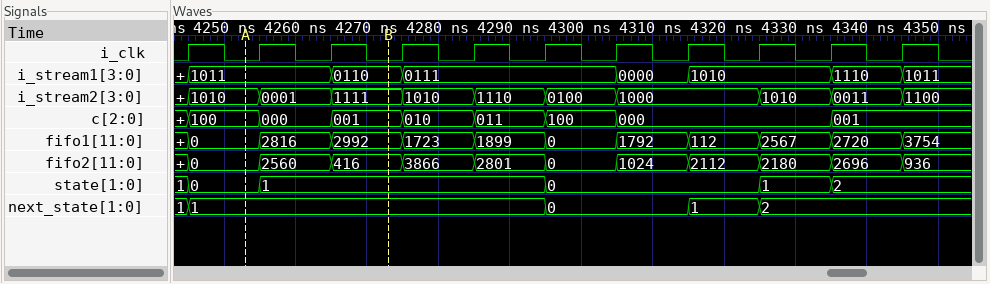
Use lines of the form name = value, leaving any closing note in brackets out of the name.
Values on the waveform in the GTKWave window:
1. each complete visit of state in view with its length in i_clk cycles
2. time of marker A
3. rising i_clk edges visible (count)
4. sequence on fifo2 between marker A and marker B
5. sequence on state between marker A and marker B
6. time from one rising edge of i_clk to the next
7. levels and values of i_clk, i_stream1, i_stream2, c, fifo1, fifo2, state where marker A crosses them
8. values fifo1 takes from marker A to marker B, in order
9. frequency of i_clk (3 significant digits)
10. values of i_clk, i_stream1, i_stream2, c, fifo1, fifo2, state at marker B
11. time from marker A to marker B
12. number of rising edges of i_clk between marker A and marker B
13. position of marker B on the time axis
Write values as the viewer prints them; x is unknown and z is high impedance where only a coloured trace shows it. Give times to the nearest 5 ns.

each complete visit of state in view with its length in i_clk cycles = 0: 1, 1: 4, 0: 3, 1: 1
time of marker A = 4255 ns
rising i_clk edges visible = 11
sequence on fifo2 between marker A and marker B = 0, 2560, 416
sequence on state between marker A and marker B = 0, 1
time from one rising edge of i_clk to the next = 10 ns
levels and values of i_clk, i_stream1, i_stream2, c, fifo1, fifo2, state where marker A crosses them = i_clk=0, i_stream1=1011, i_stream2=1010, c=100, fifo1=0, fifo2=0, state=0
values fifo1 takes from marker A to marker B, in order = 0, 2816, 2992
frequency of i_clk = 100 MHz
values of i_clk, i_stream1, i_stream2, c, fifo1, fifo2, state at marker B = i_clk=0, i_stream1=0110, i_stream2=1111, c=001, fifo1=2992, fifo2=416, state=1
time from marker A to marker B = 20 ns
number of rising edges of i_clk between marker A and marker B = 2
position of marker B on the time axis = 4275 ns
